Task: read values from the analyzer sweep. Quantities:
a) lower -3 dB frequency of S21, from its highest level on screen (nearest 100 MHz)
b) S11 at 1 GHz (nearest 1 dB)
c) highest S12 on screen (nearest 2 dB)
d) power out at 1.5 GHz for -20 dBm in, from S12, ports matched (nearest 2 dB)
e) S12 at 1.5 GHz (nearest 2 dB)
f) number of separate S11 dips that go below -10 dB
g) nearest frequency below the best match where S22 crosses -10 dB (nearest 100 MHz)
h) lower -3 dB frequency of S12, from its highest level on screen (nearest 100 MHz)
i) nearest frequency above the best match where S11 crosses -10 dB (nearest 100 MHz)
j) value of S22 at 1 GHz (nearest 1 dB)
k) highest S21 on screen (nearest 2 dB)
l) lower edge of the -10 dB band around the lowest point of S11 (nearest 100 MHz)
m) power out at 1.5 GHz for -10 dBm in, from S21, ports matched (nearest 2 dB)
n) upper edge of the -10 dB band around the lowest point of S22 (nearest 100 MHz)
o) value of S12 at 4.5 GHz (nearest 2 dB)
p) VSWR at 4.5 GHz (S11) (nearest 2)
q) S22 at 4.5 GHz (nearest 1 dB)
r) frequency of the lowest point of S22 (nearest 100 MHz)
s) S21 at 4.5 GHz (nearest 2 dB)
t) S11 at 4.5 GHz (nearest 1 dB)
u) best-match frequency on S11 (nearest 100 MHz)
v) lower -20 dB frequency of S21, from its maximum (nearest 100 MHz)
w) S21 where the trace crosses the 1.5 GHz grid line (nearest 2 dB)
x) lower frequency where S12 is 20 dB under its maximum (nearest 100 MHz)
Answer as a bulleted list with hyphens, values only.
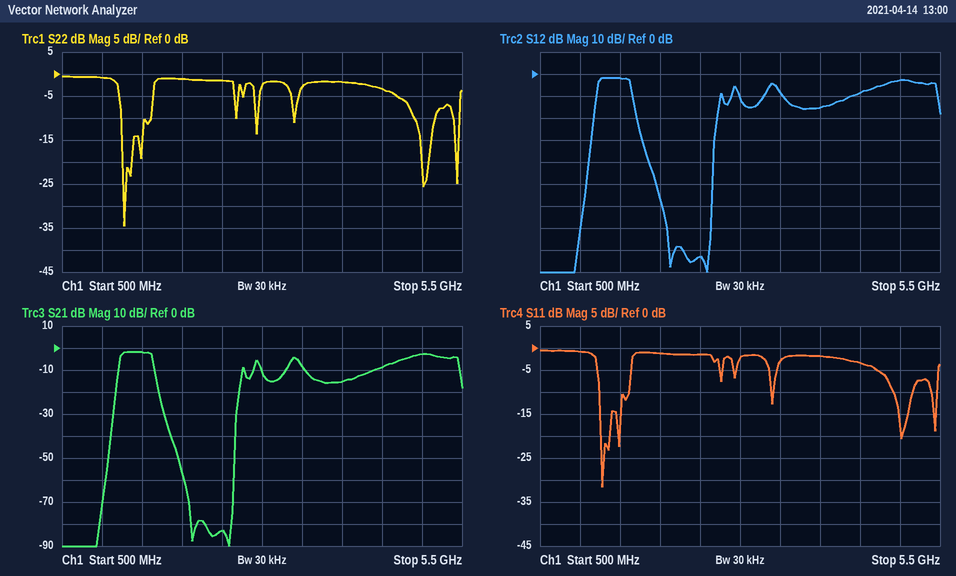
- 1.2 GHz
- -1 dB
- -2 dB
- -22 dBm
- -2 dB
- 5
- 1.2 GHz
- 1.2 GHz
- 1.6 GHz
- -1 dB
- -2 dB
- 1.2 GHz
- -12 dBm
- 1.6 GHz
- -8 dB
- 6
- -3 dB
- 1.3 GHz
- -8 dB
- -3 dB
- 1.3 GHz
- 1.2 GHz
- -2 dB
- 1.2 GHz
